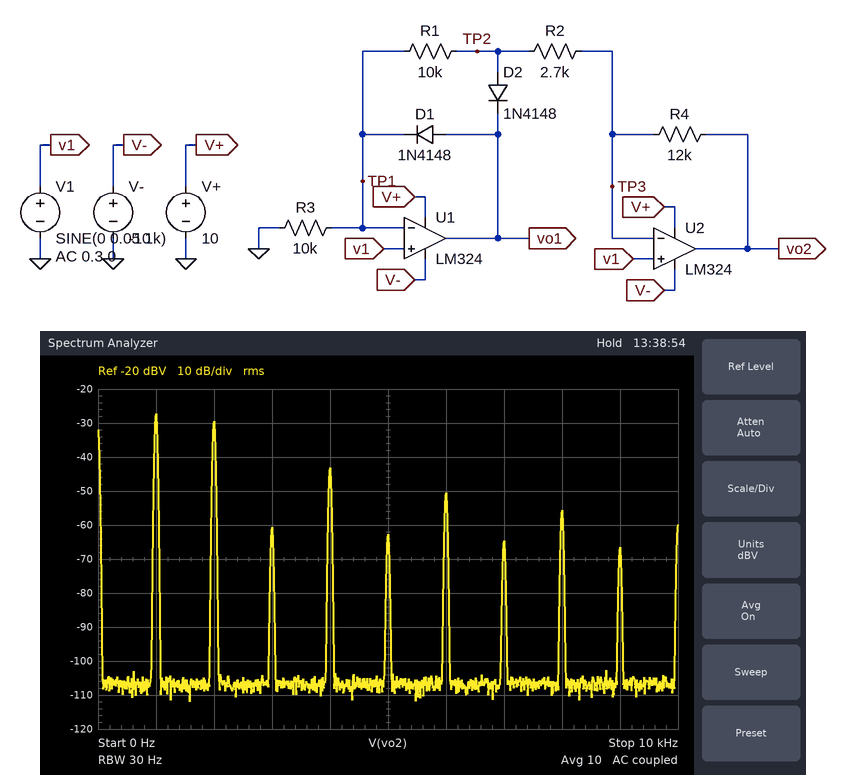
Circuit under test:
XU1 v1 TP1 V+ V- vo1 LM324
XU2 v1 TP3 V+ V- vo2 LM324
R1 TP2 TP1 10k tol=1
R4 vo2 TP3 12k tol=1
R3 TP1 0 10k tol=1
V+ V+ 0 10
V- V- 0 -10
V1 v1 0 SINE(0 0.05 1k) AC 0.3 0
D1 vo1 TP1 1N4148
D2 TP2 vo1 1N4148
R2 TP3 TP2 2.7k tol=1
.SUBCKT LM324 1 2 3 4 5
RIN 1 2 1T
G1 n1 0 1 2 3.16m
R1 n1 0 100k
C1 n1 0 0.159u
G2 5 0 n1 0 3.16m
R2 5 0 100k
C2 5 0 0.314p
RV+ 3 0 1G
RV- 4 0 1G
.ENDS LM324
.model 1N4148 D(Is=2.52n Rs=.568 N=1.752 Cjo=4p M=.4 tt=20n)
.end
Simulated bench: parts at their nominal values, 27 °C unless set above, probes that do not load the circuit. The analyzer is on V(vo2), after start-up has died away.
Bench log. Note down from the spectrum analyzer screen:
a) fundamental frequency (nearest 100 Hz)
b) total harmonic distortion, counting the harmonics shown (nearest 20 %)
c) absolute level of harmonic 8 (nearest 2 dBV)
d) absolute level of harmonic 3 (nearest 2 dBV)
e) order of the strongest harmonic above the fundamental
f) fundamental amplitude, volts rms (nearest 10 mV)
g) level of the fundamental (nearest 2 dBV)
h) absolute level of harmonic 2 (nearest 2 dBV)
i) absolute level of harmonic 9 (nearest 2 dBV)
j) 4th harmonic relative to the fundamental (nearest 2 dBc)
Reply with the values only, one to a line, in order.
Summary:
1.0 kHz
80 %
-56 dBV
-60 dBV
2
40 mV
-28 dBV
-30 dBV
-66 dBV
-16 dBc
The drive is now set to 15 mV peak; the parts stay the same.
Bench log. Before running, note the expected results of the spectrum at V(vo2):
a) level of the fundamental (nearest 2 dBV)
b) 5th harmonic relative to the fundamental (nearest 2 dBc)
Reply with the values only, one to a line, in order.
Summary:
-38 dBV
-26 dBc
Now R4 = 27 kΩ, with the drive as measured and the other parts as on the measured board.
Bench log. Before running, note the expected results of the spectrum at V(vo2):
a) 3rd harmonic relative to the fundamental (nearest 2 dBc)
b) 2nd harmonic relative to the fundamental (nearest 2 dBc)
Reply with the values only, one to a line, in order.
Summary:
-36 dBc
-6 dBc
